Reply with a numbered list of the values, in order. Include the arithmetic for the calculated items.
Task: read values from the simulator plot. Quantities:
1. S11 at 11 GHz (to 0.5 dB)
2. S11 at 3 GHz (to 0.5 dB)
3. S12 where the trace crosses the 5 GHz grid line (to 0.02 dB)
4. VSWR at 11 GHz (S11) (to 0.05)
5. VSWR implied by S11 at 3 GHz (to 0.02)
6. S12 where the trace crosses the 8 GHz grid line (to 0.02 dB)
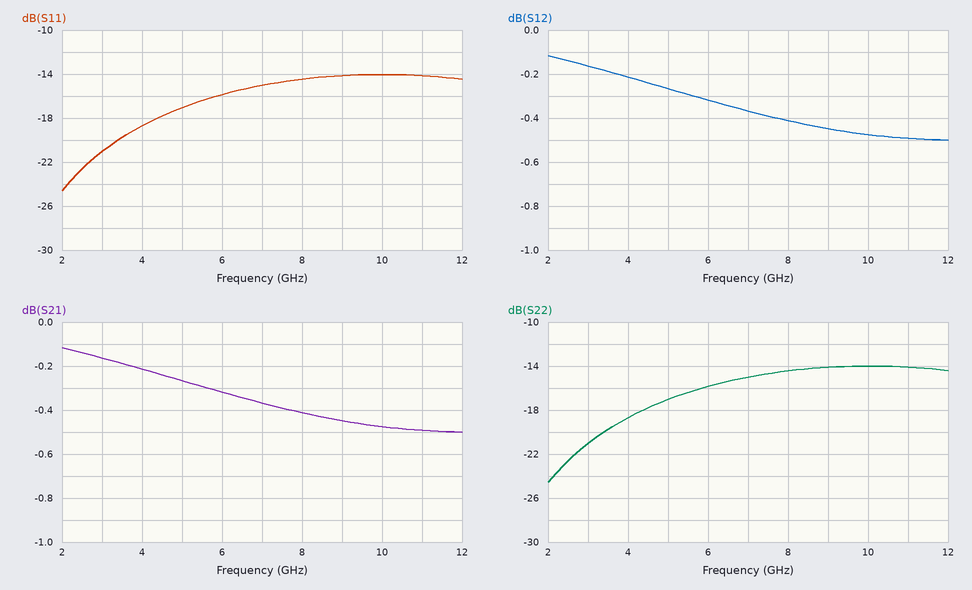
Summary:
1. -14.0 dB
2. -21.0 dB
3. -0.26 dB
4. |Γ| = 10^(-14/20) = 0.1995; VSWR = (1 + 0.1995)/(1 − 0.1995) ≈ 1.50
5. |Γ| = 10^(-21/20) = 0.0891; VSWR = (1 + 0.0891)/(1 − 0.0891) ≈ 1.20
6. -0.42 dB
